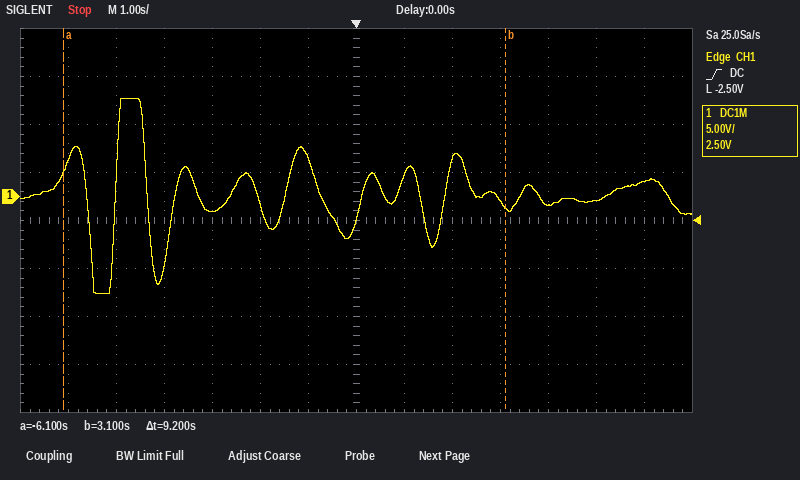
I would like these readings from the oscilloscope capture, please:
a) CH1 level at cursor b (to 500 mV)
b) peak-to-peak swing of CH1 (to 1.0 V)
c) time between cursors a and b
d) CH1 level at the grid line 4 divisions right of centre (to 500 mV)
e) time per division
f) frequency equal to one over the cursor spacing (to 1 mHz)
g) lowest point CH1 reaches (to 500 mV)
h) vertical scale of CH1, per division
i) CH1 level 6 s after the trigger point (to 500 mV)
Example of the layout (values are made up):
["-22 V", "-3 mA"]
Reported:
["-1.0 V", "20.0 V", "9.2 s", "-1.0 V", "1 s", "109 mHz", "-10.0 V", "5 V", "1.5 V"]
